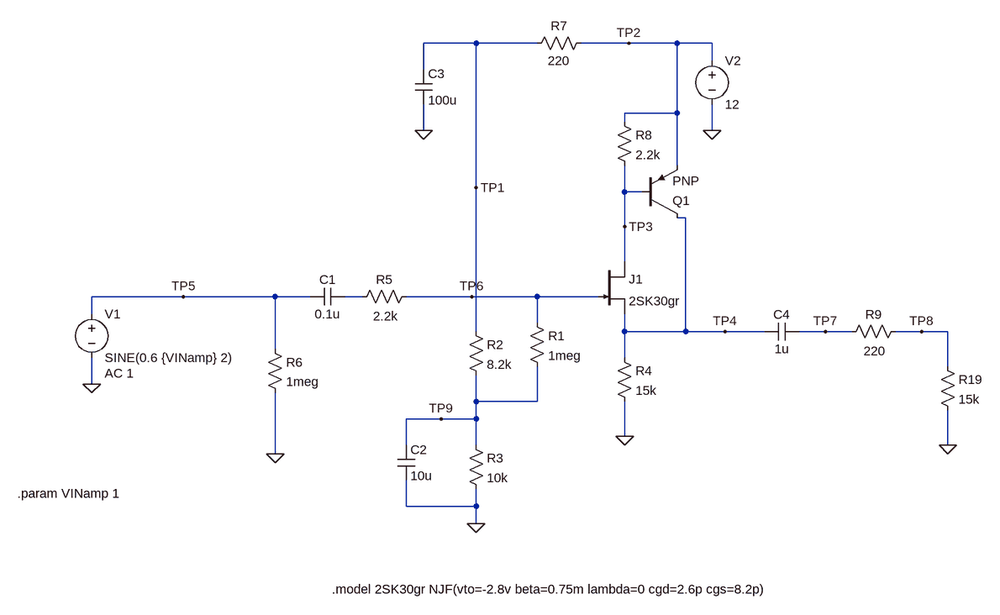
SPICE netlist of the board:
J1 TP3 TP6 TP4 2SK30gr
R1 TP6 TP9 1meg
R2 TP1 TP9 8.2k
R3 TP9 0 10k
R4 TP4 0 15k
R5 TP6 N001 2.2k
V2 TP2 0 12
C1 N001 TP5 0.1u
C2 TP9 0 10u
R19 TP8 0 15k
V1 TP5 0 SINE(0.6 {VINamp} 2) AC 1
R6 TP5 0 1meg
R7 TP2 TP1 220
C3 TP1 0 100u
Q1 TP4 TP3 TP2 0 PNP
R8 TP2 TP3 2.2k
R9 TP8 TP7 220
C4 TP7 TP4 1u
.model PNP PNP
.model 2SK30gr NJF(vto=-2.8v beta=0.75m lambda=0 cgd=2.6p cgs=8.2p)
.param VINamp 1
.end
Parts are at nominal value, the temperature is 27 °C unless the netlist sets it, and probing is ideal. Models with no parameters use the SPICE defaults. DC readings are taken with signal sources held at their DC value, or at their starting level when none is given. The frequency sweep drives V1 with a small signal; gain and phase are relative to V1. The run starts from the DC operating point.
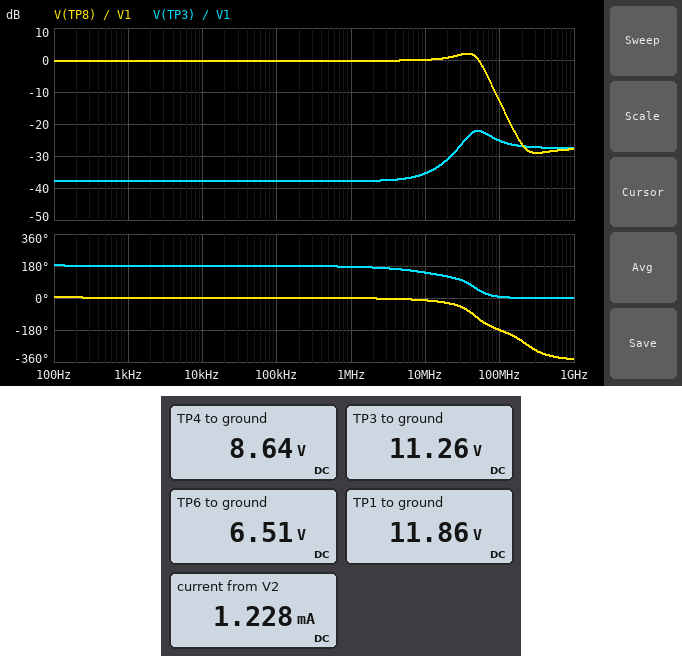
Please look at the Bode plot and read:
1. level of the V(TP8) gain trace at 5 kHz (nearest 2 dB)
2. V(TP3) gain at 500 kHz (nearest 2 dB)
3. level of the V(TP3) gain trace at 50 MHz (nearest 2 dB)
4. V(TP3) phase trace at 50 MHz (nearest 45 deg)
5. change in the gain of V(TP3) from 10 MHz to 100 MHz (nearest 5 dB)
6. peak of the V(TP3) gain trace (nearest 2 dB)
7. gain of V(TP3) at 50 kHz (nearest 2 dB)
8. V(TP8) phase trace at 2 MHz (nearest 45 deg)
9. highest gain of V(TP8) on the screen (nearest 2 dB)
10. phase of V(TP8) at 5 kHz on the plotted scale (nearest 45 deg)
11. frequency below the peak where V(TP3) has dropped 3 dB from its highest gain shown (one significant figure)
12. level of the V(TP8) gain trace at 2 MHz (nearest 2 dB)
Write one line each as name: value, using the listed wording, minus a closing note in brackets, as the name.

level of the V(TP8) gain trace at 5 kHz: 0 dB
V(TP3) gain at 500 kHz: -38 dB
level of the V(TP3) gain trace at 50 MHz: -22 dB
V(TP3) phase trace at 50 MHz: 45 deg
change in the gain of V(TP3) from 10 MHz to 100 MHz: 10 dB
peak of the V(TP3) gain trace: -22 dB
gain of V(TP3) at 50 kHz: -38 dB
V(TP8) phase trace at 2 MHz: 0 deg
highest gain of V(TP8) on the screen: 2 dB
phase of V(TP8) at 5 kHz on the plotted scale: 0 deg
frequency below the peak where V(TP3) has dropped 3 dB from its highest gain shown: 30 MHz
level of the V(TP8) gain trace at 2 MHz: 0 dB
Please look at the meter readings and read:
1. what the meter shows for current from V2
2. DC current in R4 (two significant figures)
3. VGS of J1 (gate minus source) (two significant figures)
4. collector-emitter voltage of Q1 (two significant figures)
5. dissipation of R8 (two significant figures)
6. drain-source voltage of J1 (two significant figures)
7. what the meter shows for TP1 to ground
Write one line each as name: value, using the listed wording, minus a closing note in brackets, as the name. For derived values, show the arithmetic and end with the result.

what the meter shows for current from V2: 1.228 mA
DC current in R4: (8.64 V) / 15 kΩ = 580 µA
VGS of J1 (gate minus source): 6.51 V - 8.64 V = -2.1 V
collector-emitter voltage of Q1: 8.64 V - 12 V = -3.4 V
dissipation of R8: (12 V - 11.26 V)^2 / 2.2 kΩ = 250 µW
drain-source voltage of J1: 11.26 V - 8.64 V = 2.6 V
what the meter shows for TP1 to ground: 11.86 V
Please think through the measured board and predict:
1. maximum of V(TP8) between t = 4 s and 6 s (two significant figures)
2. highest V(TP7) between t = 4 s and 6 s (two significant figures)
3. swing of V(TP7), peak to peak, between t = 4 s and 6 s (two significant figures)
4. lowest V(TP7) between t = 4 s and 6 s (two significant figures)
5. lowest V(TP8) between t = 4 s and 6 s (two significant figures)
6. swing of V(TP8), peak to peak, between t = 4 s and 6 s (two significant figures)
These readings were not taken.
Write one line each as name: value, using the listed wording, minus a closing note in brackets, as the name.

maximum of V(TP8) between t = 4 s and 6 s: 140 mV
highest V(TP7) between t = 4 s and 6 s: 150 mV
swing of V(TP7), peak to peak, between t = 4 s and 6 s: 290 mV
lowest V(TP7) between t = 4 s and 6 s: -150 mV
lowest V(TP8) between t = 4 s and 6 s: -140 mV
swing of V(TP8), peak to peak, between t = 4 s and 6 s: 290 mV
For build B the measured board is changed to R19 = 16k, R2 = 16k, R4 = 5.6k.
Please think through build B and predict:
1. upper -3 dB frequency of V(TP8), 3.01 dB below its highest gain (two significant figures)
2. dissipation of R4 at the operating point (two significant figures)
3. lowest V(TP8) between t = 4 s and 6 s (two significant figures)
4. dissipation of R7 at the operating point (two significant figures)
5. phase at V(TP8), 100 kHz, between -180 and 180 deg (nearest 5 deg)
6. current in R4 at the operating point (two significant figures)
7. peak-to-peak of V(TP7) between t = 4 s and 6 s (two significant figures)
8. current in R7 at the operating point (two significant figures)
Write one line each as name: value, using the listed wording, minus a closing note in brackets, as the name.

upper -3 dB frequency of V(TP8), 3.01 dB below its highest gain: 62 MHz
dissipation of R4 at the operating point: 8.0 mW
lowest V(TP8) between t = 4 s and 6 s: -150 mV
dissipation of R7 at the operating point: 46 µW
phase at V(TP8), 100 kHz, between -180 and 180 deg: 0 deg
current in R4 at the operating point: 1.2 mA
peak-to-peak of V(TP7) between t = 4 s and 6 s: 310 mV
current in R7 at the operating point: 460 µA
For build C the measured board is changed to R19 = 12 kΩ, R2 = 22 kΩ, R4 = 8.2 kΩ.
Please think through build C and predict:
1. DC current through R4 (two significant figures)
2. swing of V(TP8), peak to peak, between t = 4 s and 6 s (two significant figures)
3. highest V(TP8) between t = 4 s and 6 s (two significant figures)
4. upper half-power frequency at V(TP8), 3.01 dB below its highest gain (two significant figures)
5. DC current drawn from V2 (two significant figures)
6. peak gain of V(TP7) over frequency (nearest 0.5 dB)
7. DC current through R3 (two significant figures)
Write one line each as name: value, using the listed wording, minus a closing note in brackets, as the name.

DC current through R4: 710 µA
swing of V(TP8), peak to peak, between t = 4 s and 6 s: 230 mV
highest V(TP8) between t = 4 s and 6 s: 120 mV
upper half-power frequency at V(TP8), 3.01 dB below its highest gain: 62 MHz
DC current drawn from V2: 1.1 mA
peak gain of V(TP7) over frequency: 3.0 dB
DC current through R3: 370 µA
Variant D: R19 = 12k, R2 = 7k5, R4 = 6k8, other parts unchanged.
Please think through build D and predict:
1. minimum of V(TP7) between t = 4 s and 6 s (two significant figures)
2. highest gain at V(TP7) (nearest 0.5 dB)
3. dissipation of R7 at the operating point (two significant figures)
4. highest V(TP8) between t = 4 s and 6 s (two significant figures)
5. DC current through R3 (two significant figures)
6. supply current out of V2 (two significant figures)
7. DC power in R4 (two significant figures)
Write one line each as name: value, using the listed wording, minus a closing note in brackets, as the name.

minimum of V(TP7) between t = 4 s and 6 s: -120 mV
highest gain at V(TP7): 3.0 dB
dissipation of R7 at the operating point: 100 µW
highest V(TP8) between t = 4 s and 6 s: 120 mV
DC current through R3: 680 µA
supply current out of V2: 2.0 mA
DC power in R4: 12 mW
